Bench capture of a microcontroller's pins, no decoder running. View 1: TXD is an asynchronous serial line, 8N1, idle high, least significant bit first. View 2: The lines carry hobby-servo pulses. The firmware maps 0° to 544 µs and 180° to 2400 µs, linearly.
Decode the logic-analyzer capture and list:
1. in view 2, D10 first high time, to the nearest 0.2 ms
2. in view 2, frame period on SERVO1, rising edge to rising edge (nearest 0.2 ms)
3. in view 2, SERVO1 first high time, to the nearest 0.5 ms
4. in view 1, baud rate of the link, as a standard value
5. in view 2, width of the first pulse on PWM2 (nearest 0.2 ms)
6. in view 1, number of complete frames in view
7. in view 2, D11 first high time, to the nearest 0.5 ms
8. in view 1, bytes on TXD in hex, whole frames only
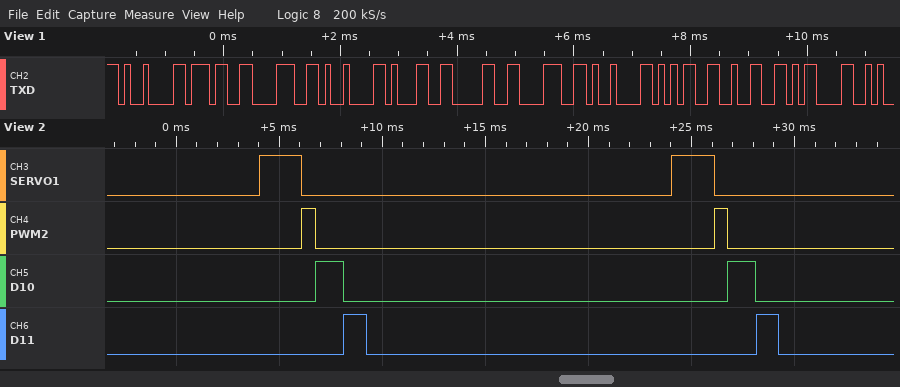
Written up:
1.4 ms
20.0 ms
2.0 ms
9600 baud
0.6 ms
11
1.0 ms
0x09 0x37 0x38 0x09 0x31 0x30 0x38 0x09 0x35 0x32 0x0D
